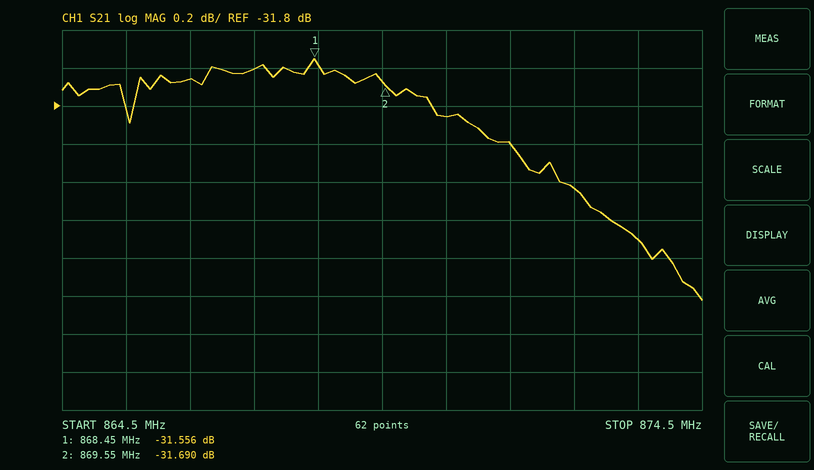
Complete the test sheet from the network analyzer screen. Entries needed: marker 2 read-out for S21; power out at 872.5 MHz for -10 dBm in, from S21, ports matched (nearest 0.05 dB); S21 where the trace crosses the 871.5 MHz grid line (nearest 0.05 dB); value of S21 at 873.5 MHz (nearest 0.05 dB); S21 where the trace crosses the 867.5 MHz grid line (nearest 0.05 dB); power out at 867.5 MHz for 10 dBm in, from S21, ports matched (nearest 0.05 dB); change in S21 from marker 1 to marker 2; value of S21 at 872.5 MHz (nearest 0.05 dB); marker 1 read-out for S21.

-31.690 dB
-42.25 dBm
-32.00 dB
-32.50 dB
-31.60 dB
-21.60 dBm
-0.134 dB
-32.25 dB
-31.556 dB
